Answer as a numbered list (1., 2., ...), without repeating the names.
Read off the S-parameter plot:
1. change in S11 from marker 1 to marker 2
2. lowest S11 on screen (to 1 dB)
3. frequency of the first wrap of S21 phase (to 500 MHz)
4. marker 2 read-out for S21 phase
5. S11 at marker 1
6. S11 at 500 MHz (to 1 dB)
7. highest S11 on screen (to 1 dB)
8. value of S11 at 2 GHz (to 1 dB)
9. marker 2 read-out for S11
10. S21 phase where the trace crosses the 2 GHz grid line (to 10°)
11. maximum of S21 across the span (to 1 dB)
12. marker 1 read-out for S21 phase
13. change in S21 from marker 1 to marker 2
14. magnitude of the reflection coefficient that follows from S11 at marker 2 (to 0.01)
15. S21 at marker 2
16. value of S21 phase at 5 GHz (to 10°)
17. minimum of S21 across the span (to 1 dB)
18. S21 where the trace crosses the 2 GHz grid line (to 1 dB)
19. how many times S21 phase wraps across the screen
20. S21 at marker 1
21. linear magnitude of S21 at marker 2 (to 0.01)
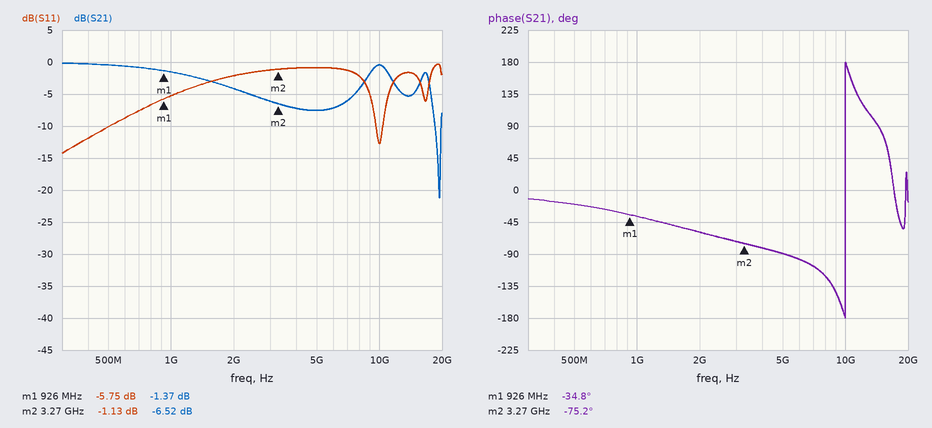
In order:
1. 4.62 dB
2. -14 dB
3. 10.0 GHz
4. -75.2°
5. -5.75 dB
6. -10 dB
7. 0 dB
8. -2 dB
9. -1.13 dB
10. -60°
11. 0 dB
12. -34.8°
13. -5.15 dB
14. 0.88
15. -6.52 dB
16. -90°
17. -21 dB
18. -4 dB
19. 1
20. -1.37 dB
21. 0.47
